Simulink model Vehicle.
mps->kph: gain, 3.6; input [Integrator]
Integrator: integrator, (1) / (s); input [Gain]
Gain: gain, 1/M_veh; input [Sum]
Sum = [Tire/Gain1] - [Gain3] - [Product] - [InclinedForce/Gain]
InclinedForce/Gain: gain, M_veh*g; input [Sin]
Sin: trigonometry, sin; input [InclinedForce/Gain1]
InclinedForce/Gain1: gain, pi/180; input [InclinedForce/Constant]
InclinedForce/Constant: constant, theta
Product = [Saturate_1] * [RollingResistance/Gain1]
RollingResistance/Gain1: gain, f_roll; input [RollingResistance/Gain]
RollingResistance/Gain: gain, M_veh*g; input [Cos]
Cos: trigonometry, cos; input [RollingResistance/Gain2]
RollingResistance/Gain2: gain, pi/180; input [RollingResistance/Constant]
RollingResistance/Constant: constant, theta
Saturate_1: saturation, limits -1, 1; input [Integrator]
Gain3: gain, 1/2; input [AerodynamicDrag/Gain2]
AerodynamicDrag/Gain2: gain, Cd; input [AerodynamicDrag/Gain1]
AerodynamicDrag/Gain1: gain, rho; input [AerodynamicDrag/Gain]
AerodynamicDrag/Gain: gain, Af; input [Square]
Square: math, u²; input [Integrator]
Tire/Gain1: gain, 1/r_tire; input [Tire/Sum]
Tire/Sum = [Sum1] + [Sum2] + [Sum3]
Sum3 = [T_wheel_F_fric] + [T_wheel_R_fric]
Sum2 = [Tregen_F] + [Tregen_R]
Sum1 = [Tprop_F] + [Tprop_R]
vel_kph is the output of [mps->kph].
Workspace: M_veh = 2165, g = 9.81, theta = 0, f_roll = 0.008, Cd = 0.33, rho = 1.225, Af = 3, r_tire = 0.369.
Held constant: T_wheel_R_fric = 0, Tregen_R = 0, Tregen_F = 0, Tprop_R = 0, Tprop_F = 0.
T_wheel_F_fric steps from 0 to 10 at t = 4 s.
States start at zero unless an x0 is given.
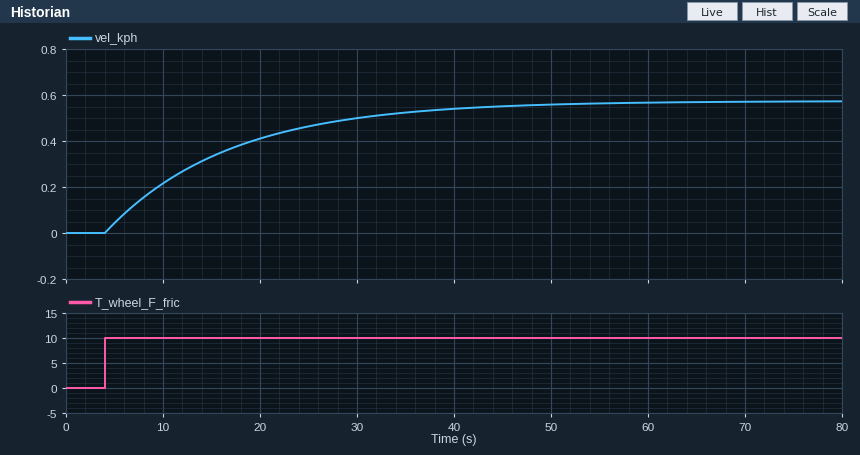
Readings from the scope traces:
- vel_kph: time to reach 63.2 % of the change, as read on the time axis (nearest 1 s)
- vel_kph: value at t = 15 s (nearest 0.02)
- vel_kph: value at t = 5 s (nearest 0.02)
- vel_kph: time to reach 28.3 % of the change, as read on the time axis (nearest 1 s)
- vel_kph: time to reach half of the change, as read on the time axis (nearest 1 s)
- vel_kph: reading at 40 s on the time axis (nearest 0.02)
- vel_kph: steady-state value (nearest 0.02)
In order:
17 s
0.34
0.04
8 s
13 s
0.54
0.58
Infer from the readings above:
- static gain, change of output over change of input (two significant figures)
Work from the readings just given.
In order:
0.058
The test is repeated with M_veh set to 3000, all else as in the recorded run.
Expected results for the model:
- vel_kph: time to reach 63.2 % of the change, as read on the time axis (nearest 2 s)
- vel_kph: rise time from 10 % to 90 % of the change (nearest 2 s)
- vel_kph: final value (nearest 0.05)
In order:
16 s
28 s
0.40
